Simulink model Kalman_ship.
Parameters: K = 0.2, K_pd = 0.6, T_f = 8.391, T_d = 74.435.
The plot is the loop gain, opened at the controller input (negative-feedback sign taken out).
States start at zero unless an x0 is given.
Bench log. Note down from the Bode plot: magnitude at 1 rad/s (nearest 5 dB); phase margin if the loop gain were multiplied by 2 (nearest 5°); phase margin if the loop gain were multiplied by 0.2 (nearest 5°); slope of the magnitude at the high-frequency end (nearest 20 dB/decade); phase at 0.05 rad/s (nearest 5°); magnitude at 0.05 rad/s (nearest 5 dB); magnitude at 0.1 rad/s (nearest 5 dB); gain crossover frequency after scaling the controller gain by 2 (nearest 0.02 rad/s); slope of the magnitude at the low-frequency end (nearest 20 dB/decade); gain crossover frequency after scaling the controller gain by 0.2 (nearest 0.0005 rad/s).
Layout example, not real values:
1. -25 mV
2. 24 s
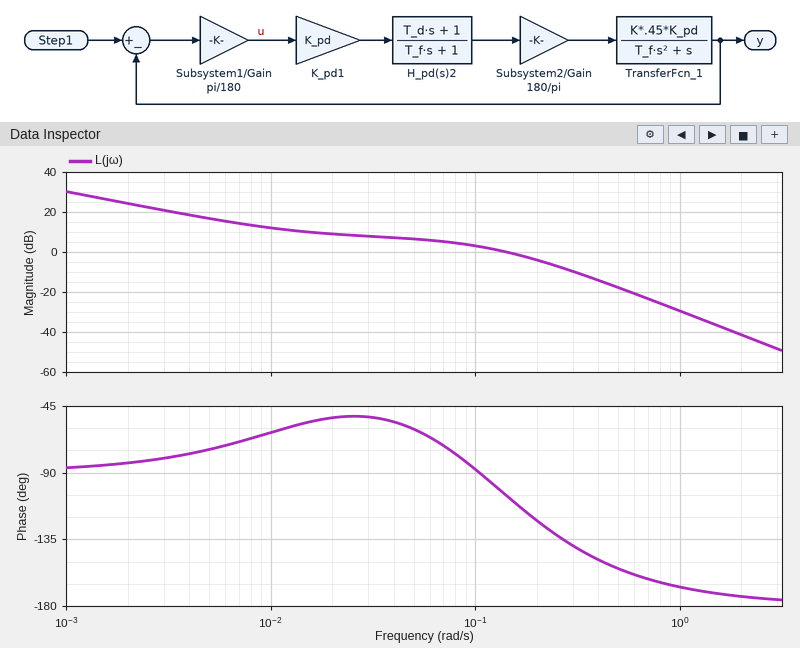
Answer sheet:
1. -30 dB
2. 50°
3. 110°
4. -40 dB/decade
5. -60°
6. 5 dB
7. 5 dB
8. 0.24 rad/s
9. -20 dB/decade
10. 0.0075 rad/s
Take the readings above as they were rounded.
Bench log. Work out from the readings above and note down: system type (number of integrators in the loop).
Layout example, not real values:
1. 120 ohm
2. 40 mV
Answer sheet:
1. 1
